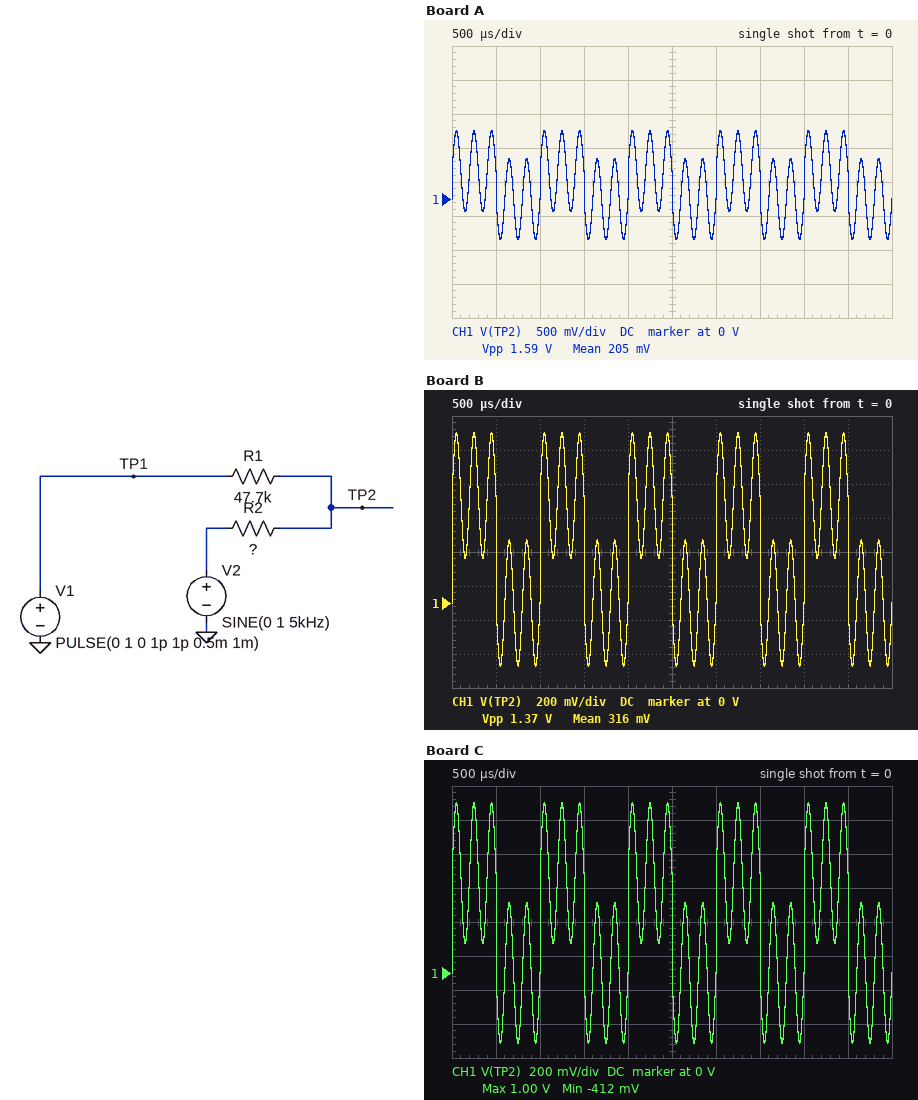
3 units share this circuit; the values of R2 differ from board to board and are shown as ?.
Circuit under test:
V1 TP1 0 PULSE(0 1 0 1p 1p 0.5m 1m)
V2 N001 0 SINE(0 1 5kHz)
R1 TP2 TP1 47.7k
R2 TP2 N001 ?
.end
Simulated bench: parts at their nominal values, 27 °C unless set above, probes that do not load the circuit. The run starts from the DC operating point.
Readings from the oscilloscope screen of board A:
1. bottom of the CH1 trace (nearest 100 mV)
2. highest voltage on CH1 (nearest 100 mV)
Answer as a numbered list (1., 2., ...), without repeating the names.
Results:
1. -600 mV
2. 1.0 V
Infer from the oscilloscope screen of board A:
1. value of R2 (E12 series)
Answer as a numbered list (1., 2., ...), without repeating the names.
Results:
1. 33 kΩ
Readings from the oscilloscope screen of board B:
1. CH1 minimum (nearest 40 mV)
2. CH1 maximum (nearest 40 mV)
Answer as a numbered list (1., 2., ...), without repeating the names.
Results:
1. -360 mV
2. 1.00 V
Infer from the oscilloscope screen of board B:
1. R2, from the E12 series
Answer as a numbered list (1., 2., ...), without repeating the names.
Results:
1. 82 kΩ
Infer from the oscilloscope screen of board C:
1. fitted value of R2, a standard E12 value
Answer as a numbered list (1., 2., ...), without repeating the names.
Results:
1. 68 kΩ
